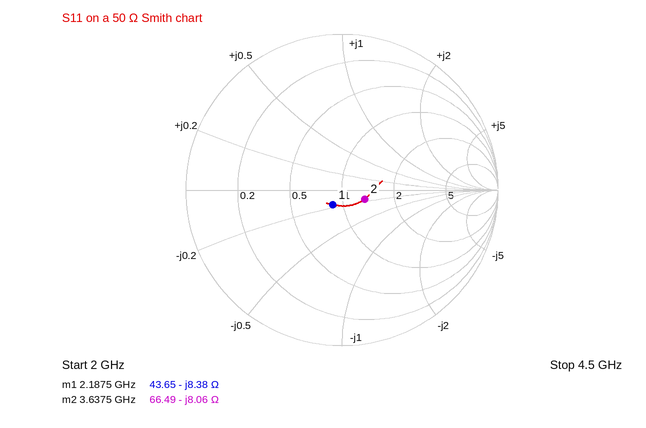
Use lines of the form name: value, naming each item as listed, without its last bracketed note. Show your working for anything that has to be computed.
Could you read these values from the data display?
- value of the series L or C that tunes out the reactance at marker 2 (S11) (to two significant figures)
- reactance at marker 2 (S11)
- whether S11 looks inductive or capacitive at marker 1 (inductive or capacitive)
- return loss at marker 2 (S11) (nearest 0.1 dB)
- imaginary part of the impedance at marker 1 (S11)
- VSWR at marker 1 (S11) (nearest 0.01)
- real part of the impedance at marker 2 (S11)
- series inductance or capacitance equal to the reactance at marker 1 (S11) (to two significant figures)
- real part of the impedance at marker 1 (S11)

value of the series L or C that tunes out the reactance at marker 2 (S11): L = 8.06 Ω/(2π × 3.6375 GHz) ≈ 353 pH, so 350 pH to two significant figures
reactance at marker 2: -8.06 Ω
whether S11 looks inductive or capacitive at marker 1: capacitive
return loss at marker 2 (S11): 16.1 dB
imaginary part of the impedance at marker 1: -8.38 Ω
VSWR at marker 1 (S11): 1.25
real part of the impedance at marker 2: 66.49 Ω
series inductance or capacitance equal to the reactance at marker 1 (S11): C = 1/(2π × 2.1875 GHz × 8.38 Ω) ≈ 8.7 pF
real part of the impedance at marker 1: 43.65 Ω
